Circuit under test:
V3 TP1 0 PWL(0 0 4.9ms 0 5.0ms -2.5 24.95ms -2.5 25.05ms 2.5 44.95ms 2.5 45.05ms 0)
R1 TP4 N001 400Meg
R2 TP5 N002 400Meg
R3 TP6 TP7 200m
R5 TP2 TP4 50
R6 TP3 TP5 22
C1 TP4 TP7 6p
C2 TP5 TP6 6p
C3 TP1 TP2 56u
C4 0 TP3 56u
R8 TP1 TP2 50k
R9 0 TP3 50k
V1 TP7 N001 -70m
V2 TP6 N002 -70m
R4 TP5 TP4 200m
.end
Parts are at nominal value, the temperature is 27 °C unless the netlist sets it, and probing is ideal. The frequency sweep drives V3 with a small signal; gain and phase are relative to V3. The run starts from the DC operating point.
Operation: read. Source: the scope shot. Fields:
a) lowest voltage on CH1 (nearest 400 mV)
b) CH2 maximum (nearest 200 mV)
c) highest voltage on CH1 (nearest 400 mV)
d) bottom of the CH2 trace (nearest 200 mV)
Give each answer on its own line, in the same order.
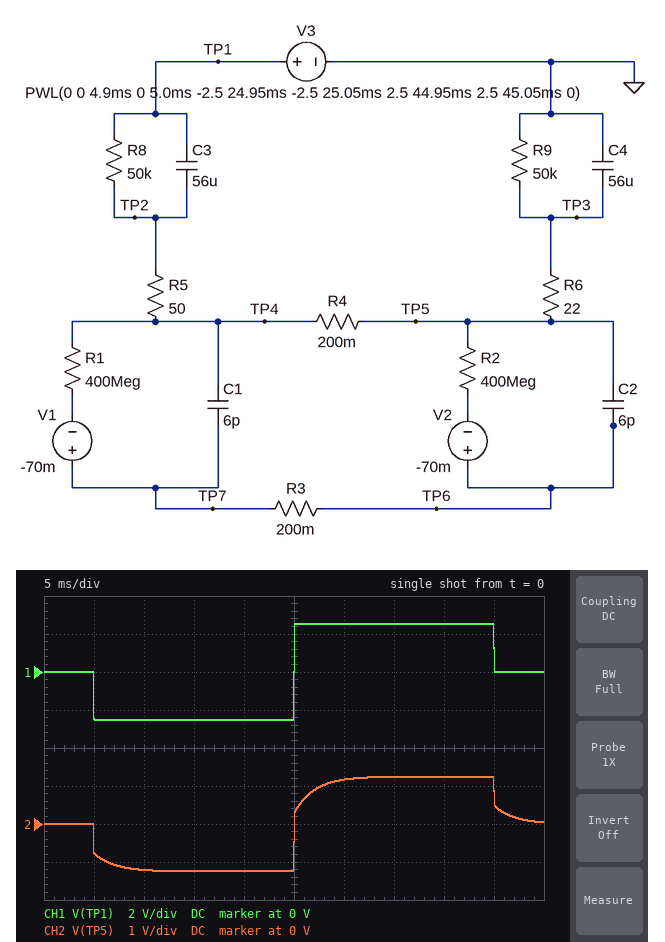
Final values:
-2.4 V
1.2 V
2.4 V
-1.2 V
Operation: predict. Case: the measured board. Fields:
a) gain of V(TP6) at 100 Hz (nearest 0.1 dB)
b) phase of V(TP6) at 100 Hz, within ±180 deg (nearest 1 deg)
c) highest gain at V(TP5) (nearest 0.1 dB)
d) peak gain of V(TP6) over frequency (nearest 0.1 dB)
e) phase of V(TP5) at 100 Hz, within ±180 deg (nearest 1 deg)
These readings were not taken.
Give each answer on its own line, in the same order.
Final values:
-8.1 dB
-14 deg
-6.0 dB
-6.0 dB
-14 deg
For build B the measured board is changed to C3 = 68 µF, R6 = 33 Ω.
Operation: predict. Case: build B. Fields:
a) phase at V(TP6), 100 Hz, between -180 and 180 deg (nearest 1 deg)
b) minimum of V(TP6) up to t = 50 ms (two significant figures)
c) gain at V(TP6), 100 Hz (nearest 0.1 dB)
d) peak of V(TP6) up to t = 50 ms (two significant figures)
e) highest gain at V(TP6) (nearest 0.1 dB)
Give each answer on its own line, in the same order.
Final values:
-9 deg
-1.4 V
-7.0 dB
1.3 V
-5.2 dB
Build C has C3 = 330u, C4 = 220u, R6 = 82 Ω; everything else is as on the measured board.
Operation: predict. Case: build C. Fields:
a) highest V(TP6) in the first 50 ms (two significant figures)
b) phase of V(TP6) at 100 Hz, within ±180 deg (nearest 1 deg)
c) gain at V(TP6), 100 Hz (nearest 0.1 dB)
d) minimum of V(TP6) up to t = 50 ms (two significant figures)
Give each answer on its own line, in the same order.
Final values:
1.5 V
0 deg
-4.1 dB
-1.6 V
